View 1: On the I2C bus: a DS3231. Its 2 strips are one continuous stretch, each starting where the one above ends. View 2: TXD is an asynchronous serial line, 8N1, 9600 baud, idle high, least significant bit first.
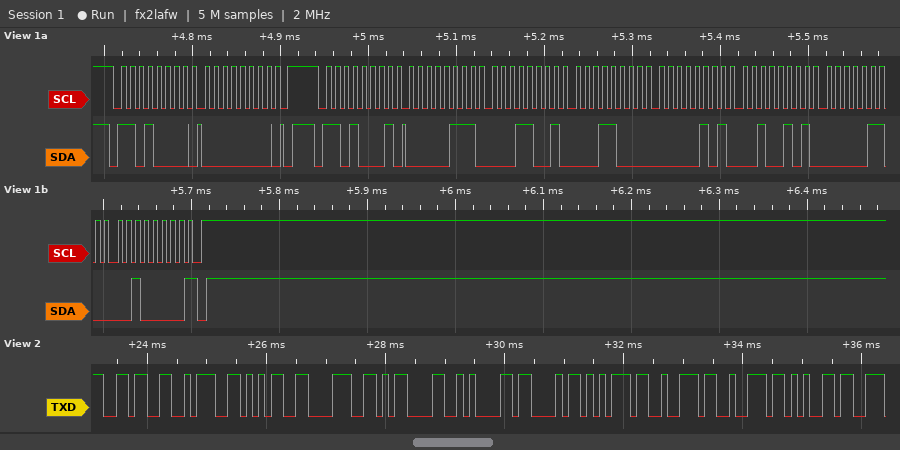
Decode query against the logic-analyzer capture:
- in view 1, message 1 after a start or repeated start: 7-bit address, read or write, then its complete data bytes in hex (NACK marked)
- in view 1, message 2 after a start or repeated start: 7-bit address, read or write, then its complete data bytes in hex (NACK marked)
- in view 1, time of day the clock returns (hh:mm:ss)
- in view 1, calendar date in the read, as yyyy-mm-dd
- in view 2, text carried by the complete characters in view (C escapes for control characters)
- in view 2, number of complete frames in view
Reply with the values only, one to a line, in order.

0x68 write: 00
0x68 read: 07 19 18 05 25 06 20 NACK
18:19:07
2020-06-25
"6:58\r\nCurre"
11
